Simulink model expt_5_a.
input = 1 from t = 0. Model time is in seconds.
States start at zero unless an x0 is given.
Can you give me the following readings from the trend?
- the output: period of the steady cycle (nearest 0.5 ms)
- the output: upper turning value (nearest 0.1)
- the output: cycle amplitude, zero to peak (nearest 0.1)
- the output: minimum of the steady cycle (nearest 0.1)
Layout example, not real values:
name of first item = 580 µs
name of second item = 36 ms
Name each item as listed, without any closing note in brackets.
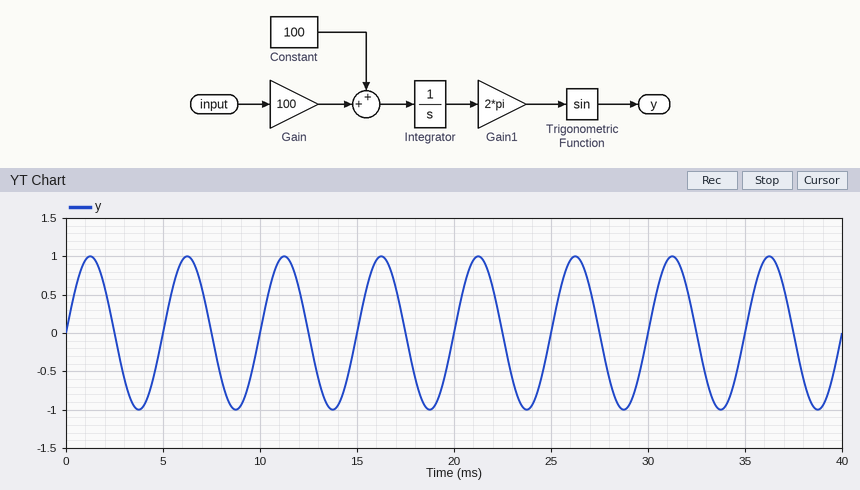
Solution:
the output: period of the steady cycle = 5.0 ms
the output: upper turning value = 1.0
the output: cycle amplitude, zero to peak = 1.0
the output: minimum of the steady cycle = -1.0
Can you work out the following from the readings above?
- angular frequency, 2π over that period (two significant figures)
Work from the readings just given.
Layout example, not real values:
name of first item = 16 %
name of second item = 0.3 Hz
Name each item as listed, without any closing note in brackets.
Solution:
angular frequency, 2π over that period = 1.3 rad/ms
